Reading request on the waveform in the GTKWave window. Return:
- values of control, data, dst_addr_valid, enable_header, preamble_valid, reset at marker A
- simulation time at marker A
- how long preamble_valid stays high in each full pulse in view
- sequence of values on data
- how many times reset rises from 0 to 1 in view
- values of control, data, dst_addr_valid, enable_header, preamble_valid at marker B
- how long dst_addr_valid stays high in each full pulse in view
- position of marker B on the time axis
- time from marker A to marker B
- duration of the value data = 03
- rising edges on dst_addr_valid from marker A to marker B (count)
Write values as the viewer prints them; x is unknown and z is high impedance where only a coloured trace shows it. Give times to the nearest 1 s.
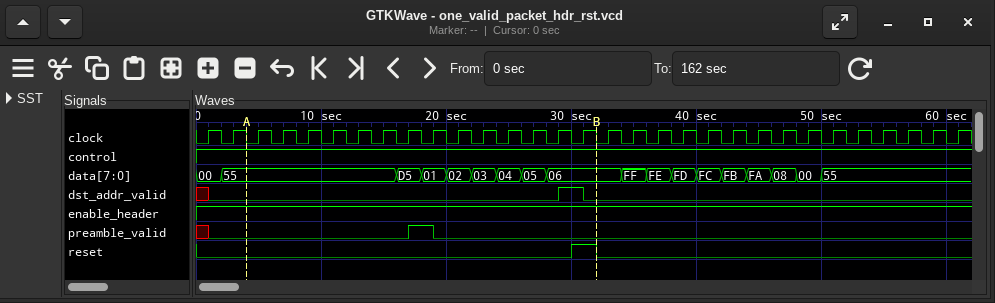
control=1, data=55, dst_addr_valid=0, enable_header=1, preamble_valid=0, reset=0
4 s
2 s
00, 55, D5, 01, 02, 03, 04, 05, 06, FF, FE, FD, FC, FB, FA, 08, 00, 55
1
control=1, data=06, dst_addr_valid=0, enable_header=1, preamble_valid=0
2 s
32 s
28 s
2 s
1
